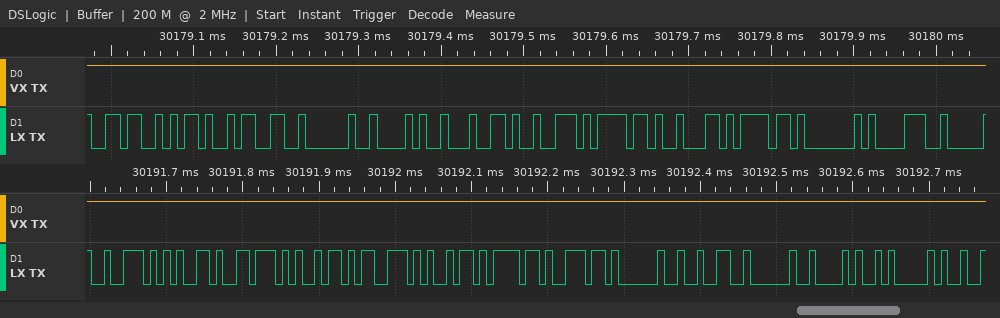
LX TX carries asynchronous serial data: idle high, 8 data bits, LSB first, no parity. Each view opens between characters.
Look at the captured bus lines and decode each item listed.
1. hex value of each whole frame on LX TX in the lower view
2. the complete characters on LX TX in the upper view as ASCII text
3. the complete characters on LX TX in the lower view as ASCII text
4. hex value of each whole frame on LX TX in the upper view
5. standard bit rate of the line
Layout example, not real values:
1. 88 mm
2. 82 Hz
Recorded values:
1. 72, 65, 76, 69, 73, 69, 6F, 6E, 20, 32, 20, 28, 41
2. "6-3 (drobo@8"
3. "revision 2 (A"
4. 36, 2D, 33, 20, 28, 64, 72, 6F, 62, 6F, 40, 38
5. 115200 baud
